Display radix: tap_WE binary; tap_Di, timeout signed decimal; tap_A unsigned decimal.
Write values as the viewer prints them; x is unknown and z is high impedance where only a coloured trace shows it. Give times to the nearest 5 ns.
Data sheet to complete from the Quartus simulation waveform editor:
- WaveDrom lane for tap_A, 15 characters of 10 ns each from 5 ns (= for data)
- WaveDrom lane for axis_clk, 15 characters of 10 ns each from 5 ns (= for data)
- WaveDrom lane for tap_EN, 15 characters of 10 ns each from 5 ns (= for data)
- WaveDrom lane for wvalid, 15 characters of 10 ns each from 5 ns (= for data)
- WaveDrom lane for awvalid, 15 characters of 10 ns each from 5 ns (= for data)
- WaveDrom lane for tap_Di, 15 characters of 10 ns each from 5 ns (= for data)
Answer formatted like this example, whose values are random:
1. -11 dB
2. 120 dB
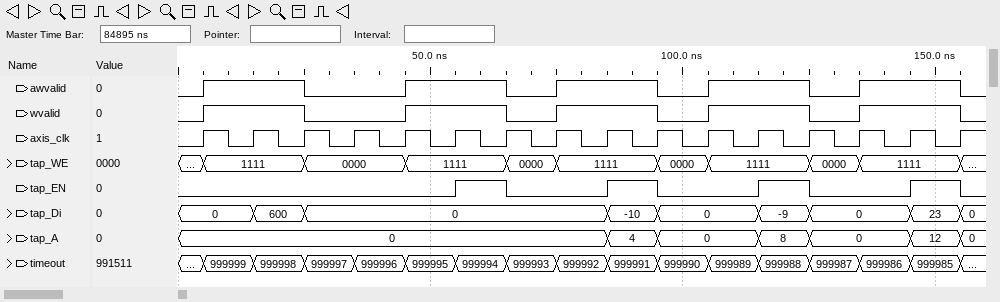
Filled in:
1. {name: 'tap_A', wave: '=.......==.==.=', data: '0 4 0 8 0 12'}
2. {name: 'axis_clk', wave: 'p..............'}
3. {name: 'tap_EN', wave: '0....10.10.10.1'}
4. {name: 'wvalid', wave: '1.0.1.01.01.01.'}
5. {name: 'awvalid', wave: '1.0.1.01.01.01.'}
6. {name: 'tap_Di', wave: '===.....==.==.=', data: '0 600 0 -10 0 -9 0 23'}
